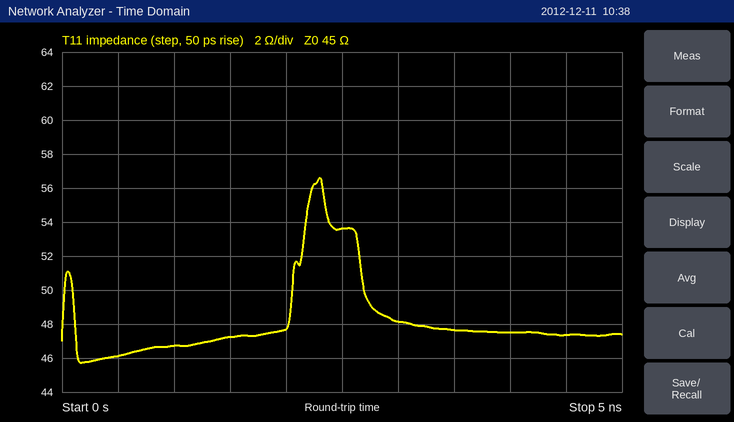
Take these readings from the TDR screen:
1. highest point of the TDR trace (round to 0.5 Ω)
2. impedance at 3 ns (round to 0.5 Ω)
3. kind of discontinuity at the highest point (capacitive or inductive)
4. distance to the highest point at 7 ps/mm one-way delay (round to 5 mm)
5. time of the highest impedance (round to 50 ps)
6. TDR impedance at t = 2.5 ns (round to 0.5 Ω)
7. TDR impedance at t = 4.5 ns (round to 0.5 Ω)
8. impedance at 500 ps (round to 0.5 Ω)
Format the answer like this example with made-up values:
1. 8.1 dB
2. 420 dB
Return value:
1. 56.5 Ω
2. 48.0 Ω
3. inductive
4. 165 mm
5. 2.30 ns
6. 53.5 Ω
7. 47.5 Ω
8. 46.0 Ω
